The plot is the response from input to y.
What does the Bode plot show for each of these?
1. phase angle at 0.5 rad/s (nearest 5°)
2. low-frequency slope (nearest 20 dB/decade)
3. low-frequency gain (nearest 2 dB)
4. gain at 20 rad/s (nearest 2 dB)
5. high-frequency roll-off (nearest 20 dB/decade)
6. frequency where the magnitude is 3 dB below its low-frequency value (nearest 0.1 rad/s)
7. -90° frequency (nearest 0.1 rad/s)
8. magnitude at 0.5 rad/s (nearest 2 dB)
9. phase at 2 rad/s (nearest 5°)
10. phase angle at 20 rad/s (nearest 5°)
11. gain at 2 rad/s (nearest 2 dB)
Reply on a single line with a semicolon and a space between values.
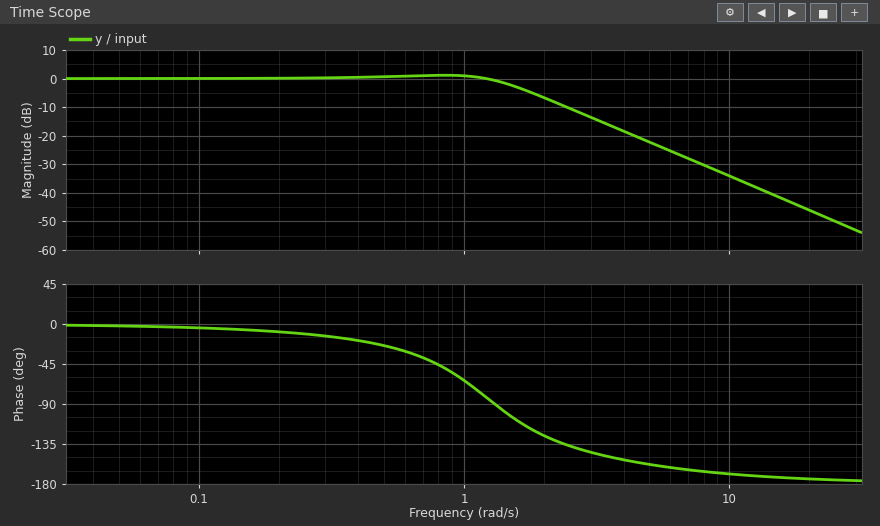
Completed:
-25°; 0 dB/decade; 0 dB; -46 dB; -40 dB/decade; 1.6 rad/s; 1.3 rad/s; 0 dB; -125°; -175°; -6 dB
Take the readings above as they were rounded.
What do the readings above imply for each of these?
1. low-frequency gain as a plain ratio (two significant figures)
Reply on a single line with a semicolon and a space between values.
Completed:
1.0
